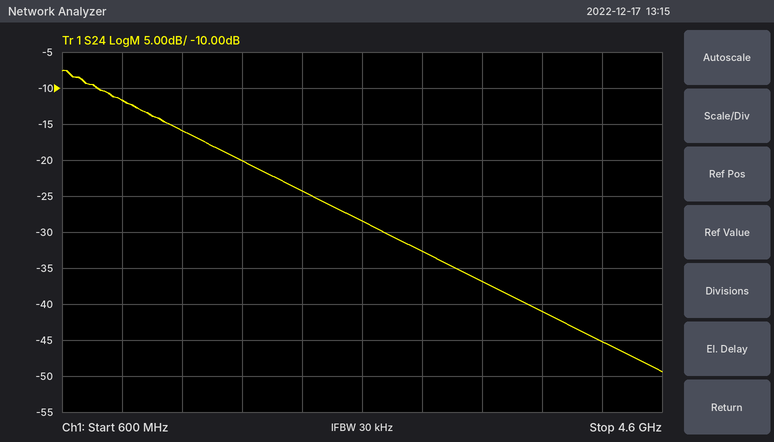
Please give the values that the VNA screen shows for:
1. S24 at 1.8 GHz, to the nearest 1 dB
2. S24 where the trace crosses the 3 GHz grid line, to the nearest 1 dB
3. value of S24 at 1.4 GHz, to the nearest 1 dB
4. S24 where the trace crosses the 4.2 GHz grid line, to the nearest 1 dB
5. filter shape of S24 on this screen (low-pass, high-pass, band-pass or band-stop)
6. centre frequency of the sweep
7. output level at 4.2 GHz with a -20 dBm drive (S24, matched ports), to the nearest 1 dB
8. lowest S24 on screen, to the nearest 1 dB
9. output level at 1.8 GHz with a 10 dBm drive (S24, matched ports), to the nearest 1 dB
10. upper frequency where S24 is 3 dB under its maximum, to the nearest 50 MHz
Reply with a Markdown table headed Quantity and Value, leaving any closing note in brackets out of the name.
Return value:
| Quantity | Value |
|---|---|
| S24 at 1.8 GHz, to the nearest 1 dB | -20 dB |
| S24 where the trace crosses the 3 GHz grid line, to the nearest 1 dB | -33 dB |
| value of S24 at 1.4 GHz, to the nearest 1 dB | -16 dB |
| S24 where the trace crosses the 4.2 GHz grid line, to the nearest 1 dB | -45 dB |
| filter shape of S24 on this screen | low-pass |
| centre frequency of the sweep | 2.6 GHz |
| output level at 4.2 GHz with a -20 dBm drive (S24, matched ports), to the nearest 1 dB | -65 dBm |
| lowest S24 on screen, to the nearest 1 dB | -49 dB |
| output level at 1.8 GHz with a 10 dBm drive (S24, matched ports), to the nearest 1 dB | -10 dBm |
| upper frequency where S24 is 3 dB under its maximum, to the nearest 50 MHz | 900 MHz |
